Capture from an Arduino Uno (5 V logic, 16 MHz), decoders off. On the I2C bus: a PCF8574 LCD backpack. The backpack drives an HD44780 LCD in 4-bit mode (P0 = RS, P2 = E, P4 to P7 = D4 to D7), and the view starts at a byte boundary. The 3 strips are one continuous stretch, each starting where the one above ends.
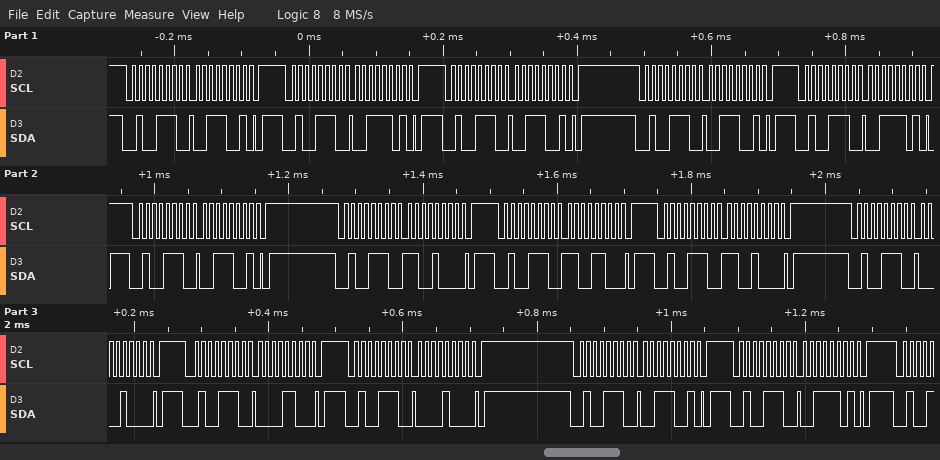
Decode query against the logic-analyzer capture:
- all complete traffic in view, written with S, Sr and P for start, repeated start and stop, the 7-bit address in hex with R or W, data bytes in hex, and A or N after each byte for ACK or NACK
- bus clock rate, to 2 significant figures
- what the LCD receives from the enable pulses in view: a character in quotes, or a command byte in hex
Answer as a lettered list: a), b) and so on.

a) S 27W A 39 A P S 27W A 3D A P S 27W A 39 A P S 27W A 39 A P S 27W A 3D A P S 27W A 39 A P S 27W A C8 A P S 27W A CC A P S 27W A C8 A P S 27W A 08 A P S 27W A 0C A P S 27W A 08 A P S 27W A 39 A P S 27W A 3D A P
b) 100 kHz
c) '3' 0xC0
